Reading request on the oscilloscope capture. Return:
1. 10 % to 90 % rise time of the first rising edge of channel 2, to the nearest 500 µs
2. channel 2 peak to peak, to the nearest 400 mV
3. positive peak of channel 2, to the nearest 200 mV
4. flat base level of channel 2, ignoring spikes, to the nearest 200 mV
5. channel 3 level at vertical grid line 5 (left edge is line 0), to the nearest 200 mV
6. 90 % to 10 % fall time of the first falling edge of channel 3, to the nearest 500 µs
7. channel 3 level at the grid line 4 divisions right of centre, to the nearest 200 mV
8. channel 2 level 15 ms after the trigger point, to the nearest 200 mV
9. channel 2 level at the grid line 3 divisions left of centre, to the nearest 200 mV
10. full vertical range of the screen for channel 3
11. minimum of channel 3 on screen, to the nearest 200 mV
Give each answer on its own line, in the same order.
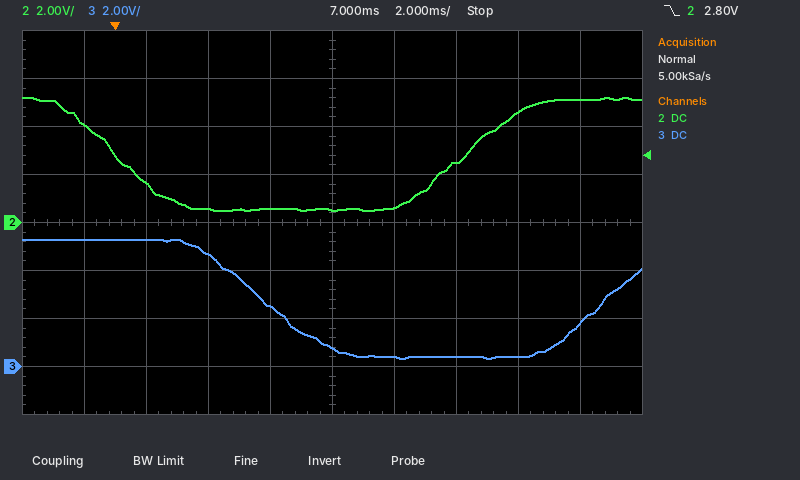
3.5 ms
4.8 V
5.2 V
600 mV
800 mV
4.0 ms
1.8 V
5.2 V
1.6 V
16 V
400 mV
